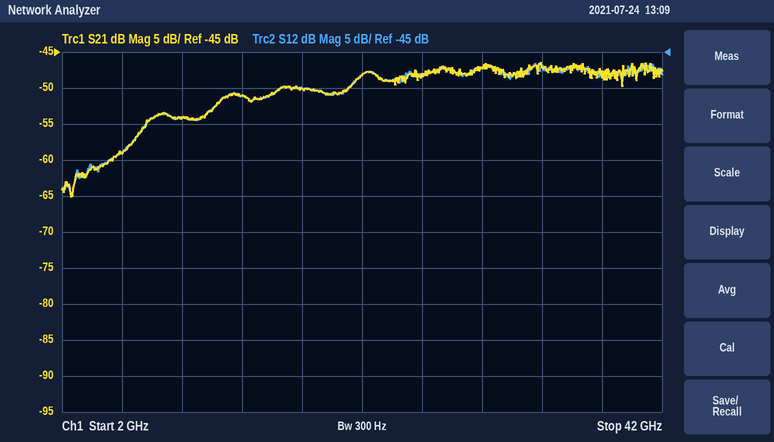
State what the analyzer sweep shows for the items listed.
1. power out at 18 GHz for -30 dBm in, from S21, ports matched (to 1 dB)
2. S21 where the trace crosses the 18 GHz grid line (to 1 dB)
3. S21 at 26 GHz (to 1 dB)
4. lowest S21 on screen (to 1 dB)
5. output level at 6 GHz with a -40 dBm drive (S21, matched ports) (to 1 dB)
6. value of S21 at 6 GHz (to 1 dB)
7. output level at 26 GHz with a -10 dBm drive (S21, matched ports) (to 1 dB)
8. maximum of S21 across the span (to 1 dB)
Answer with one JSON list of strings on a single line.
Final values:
["-80 dBm", "-50 dB", "-48 dB", "-65 dB", "-99 dBm", "-59 dB", "-58 dBm", "-46 dB"]
